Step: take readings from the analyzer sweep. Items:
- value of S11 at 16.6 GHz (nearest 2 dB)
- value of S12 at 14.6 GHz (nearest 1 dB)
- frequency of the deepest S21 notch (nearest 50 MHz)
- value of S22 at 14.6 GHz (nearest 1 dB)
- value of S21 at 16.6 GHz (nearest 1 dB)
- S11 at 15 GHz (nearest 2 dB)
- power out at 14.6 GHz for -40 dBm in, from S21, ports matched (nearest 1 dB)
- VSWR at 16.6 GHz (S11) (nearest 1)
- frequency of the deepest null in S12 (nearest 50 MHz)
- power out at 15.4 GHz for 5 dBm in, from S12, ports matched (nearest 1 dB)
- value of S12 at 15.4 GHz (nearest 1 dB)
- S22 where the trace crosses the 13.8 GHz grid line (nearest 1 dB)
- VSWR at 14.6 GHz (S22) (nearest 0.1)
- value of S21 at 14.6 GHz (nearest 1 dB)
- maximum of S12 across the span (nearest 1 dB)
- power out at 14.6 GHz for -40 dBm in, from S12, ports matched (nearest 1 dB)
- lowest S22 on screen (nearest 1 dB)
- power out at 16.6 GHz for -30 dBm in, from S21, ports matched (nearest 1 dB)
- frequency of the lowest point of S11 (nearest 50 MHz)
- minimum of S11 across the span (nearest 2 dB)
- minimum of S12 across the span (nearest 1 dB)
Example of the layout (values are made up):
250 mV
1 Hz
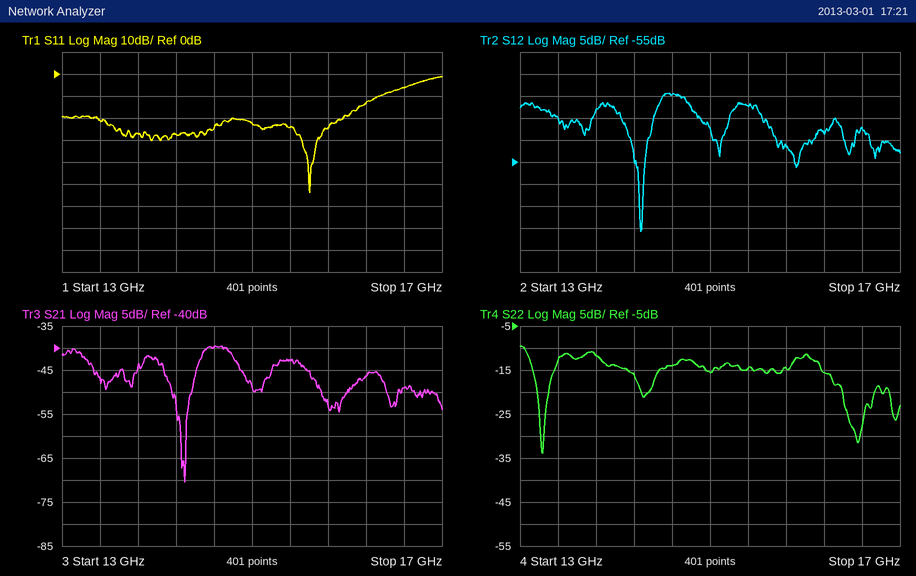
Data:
-6 dB
-40 dB
14.30 GHz
-14 dB
-49 dB
-22 dB
-80 dBm
3
14.25 GHz
-37 dBm
-42 dB
-12 dB
1.5
-40 dB
-39 dB
-80 dBm
-34 dB
-79 dBm
15.60 GHz
-54 dB
-71 dB
